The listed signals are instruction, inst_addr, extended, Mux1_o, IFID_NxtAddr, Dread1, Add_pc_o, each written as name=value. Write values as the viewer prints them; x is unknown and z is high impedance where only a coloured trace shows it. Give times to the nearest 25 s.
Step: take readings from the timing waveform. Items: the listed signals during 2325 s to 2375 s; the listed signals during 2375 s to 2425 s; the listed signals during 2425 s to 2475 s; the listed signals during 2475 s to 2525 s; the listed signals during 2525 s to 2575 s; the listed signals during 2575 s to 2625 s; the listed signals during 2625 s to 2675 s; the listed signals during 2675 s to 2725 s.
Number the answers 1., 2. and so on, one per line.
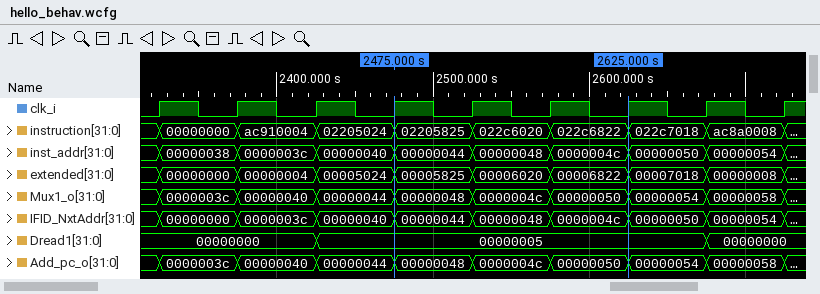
1. instruction=00000000, inst_addr=00000038, extended=00000000, Mux1_o=0000003c, IFID_NxtAddr=00000000, Dread1=00000000, Add_pc_o=0000003c
2. instruction=ac910004, inst_addr=0000003c, extended=00000004, Mux1_o=00000040, IFID_NxtAddr=0000003c, Dread1=00000000, Add_pc_o=00000040
3. instruction=02205024, inst_addr=00000040, extended=00005024, Mux1_o=00000044, IFID_NxtAddr=00000040, Dread1=00000005, Add_pc_o=00000044
4. instruction=02205825, inst_addr=00000044, extended=00005825, Mux1_o=00000048, IFID_NxtAddr=00000044, Dread1=00000005, Add_pc_o=00000048
5. instruction=022c6020, inst_addr=00000048, extended=00006020, Mux1_o=0000004c, IFID_NxtAddr=00000048, Dread1=00000005, Add_pc_o=0000004c
6. instruction=022c6822, inst_addr=0000004c, extended=00006822, Mux1_o=00000050, IFID_NxtAddr=0000004c, Dread1=00000005, Add_pc_o=00000050
7. instruction=022c7018, inst_addr=00000050, extended=00007018, Mux1_o=00000054, IFID_NxtAddr=00000050, Dread1=00000005, Add_pc_o=00000054
8. instruction=ac8a0008, inst_addr=00000054, extended=00000008, Mux1_o=00000058, IFID_NxtAddr=00000054, Dread1=00000000, Add_pc_o=00000058
